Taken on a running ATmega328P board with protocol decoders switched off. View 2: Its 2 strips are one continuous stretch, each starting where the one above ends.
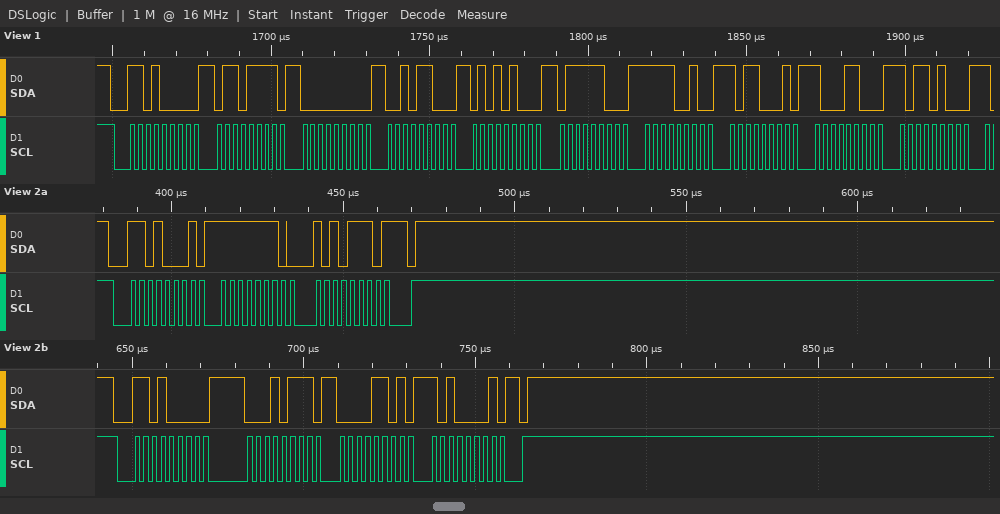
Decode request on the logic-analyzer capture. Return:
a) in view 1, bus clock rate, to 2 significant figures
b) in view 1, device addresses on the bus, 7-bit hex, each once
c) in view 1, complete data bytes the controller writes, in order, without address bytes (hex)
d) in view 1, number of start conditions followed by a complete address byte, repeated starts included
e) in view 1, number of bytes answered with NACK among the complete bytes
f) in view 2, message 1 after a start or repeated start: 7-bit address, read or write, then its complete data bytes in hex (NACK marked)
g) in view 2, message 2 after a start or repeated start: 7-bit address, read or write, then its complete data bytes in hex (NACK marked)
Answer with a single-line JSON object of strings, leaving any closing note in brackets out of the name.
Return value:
{"in view 1, bus clock rate, to 2 significant figures": "400 kHz", "in view 1, device addresses on the bus, 7-bit hex, each once": "0x68", "in view 1, complete data bytes the controller writes, in order, without address bytes": "6F 00 2C 54 7C F2 B1 8C B4", "in view 1, number of start conditions followed by a complete address byte, repeated starts included": "1", "in view 1, number of bytes answered with NACK among the complete bytes": "0", "in view 2, message 1 after a start or repeated start: 7-bit address, read or write, then its complete data bytes in hex": "0x68 read: FE AE NACK", "in view 2, message 2 after a start or repeated start: 7-bit address, read or write, then its complete data bytes in hex": "0x68 write: 17 0D A1"}
